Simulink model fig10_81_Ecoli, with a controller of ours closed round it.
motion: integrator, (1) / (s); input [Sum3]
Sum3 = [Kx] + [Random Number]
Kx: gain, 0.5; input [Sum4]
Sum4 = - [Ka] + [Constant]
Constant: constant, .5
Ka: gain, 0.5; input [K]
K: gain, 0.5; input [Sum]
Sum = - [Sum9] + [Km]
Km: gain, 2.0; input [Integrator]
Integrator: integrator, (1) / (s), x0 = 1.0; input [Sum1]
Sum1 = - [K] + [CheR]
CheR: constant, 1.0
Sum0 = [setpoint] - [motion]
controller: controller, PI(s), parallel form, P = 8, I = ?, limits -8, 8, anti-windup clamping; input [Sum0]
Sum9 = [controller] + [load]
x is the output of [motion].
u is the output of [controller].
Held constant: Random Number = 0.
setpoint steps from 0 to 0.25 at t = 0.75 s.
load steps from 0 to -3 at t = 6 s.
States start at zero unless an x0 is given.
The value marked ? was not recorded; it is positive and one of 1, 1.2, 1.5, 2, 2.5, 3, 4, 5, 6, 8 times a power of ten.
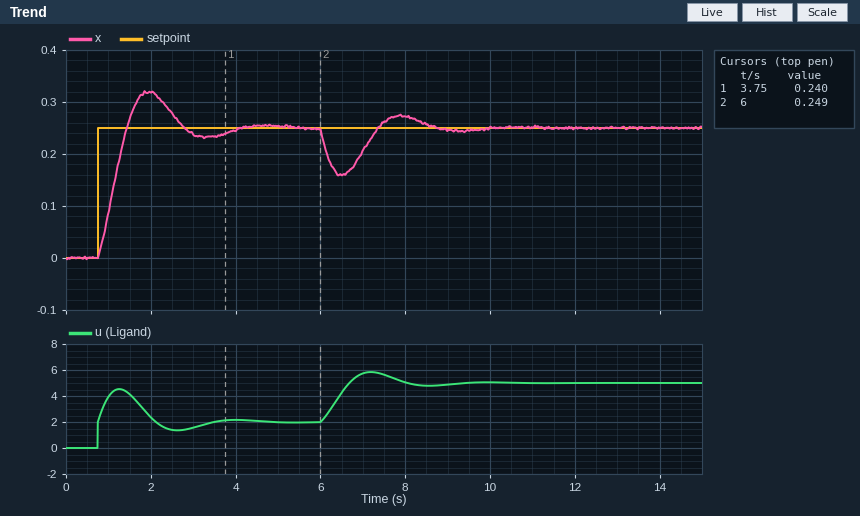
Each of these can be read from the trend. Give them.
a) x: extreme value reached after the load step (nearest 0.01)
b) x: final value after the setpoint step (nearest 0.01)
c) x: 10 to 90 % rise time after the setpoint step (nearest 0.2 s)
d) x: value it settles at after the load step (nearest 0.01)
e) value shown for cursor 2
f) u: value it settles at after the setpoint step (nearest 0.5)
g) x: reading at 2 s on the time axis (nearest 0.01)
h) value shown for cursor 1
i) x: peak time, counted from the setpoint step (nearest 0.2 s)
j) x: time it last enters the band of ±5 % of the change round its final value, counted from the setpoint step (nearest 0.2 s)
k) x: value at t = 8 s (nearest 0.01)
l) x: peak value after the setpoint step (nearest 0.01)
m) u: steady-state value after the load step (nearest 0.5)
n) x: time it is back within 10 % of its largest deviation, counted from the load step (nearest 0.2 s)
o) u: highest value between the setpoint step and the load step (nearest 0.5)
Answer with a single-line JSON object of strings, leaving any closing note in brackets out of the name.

{"x: extreme value reached after the load step": "0.16", "x: final value after the setpoint step": "0.25", "x: 10 to 90 % rise time after the setpoint step": "0.6 s", "x: value it settles at after the load step": "0.25", "value shown for cursor 2": "0.249", "u: value it settles at after the setpoint step": "2.0", "x: reading at 2 s on the time axis": "0.32", "value shown for cursor 1": "0.240", "x: peak time, counted from the setpoint step": "1.2 s", "x: time it last enters the band of ±5 % of the change round its final value, counted from the setpoint step": "3.0 s", "x: value at t = 8 s": "0.27", "x: peak value after the setpoint step": "0.32", "u: steady-state value after the load step": "5.0", "x: time it is back within 10 % of its largest deviation, counted from the load step": "2.4 s", "u: highest value between the setpoint step and the load step": "4.5"}
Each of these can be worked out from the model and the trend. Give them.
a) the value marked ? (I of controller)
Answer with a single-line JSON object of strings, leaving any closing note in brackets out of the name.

{"the value marked ?": "50"}
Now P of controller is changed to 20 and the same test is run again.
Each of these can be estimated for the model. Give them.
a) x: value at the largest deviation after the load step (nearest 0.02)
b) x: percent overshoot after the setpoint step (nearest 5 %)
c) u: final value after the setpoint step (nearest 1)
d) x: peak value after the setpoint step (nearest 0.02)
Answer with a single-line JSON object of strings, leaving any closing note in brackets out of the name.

{"x: value at the largest deviation after the load step": "0.18", "x: percent overshoot after the setpoint step": "10 %", "u: final value after the setpoint step": "2", "x: peak value after the setpoint step": "0.28"}
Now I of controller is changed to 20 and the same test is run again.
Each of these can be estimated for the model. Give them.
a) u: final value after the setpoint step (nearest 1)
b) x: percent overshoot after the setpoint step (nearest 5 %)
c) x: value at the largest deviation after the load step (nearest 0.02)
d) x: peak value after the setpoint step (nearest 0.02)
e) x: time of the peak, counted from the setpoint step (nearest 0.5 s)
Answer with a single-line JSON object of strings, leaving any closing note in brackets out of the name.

{"u: final value after the setpoint step": "2", "x: percent overshoot after the setpoint step": "10 %", "x: value at the largest deviation after the load step": "0.14", "x: peak value after the setpoint step": "0.28", "x: time of the peak, counted from the setpoint step": "2.0 s"}
